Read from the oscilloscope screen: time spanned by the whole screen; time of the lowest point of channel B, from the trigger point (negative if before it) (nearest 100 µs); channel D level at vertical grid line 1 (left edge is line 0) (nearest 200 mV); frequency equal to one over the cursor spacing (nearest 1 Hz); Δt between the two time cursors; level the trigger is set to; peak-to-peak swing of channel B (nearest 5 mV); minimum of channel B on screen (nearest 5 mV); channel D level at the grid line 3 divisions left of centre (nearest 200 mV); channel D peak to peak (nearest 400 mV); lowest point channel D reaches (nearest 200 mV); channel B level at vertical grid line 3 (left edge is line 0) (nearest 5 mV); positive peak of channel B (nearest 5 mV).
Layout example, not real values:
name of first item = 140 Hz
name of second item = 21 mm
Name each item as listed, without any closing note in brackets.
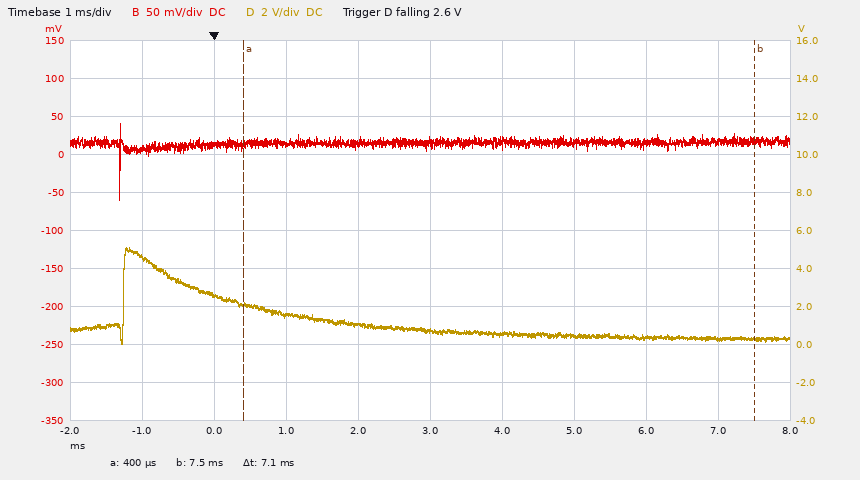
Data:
time spanned by the whole screen = 10 ms
time of the lowest point of channel B, from the trigger point (negative if before it) = -1.3 ms
channel D level at vertical grid line 1 (left edge is line 0) = 4.6 V
frequency equal to one over the cursor spacing = 141 Hz
Δt between the two time cursors = 7.1 ms
level the trigger is set to = 2.6 V
peak-to-peak swing of channel B = 100 mV
minimum of channel B on screen = -60 mV
channel D level at the grid line 3 divisions left of centre = 2.6 V
channel D peak to peak = 5.2 V
lowest point channel D reaches = 0.0 V
channel B level at vertical grid line 3 (left edge is line 0) = 15 mV
positive peak of channel B = 40 mV
